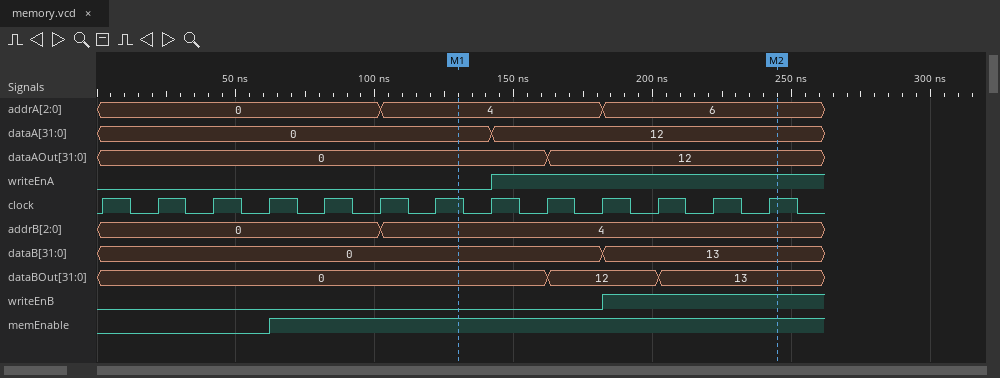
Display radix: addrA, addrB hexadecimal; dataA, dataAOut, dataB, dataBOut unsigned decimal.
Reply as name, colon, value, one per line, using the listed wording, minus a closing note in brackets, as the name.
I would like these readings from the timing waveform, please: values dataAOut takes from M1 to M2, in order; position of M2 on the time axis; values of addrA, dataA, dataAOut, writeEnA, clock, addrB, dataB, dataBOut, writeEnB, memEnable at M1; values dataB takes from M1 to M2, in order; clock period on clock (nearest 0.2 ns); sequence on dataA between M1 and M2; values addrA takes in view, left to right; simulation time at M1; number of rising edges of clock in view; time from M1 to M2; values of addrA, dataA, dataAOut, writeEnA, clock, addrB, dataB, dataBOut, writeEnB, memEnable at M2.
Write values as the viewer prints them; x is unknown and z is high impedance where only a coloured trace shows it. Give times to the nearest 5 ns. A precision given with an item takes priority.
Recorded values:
values dataAOut takes from M1 to M2, in order: 0, 12
position of M2 on the time axis: 245 ns
values of addrA, dataA, dataAOut, writeEnA, clock, addrB, dataB, dataBOut, writeEnB, memEnable at M1: addrA=4, dataA=0, dataAOut=0, writeEnA=0, clock=1, addrB=4, dataB=0, dataBOut=0, writeEnB=0, memEnable=1
values dataB takes from M1 to M2, in order: 0, 13
clock period on clock: 20 ns
sequence on dataA between M1 and M2: 0, 12
values addrA takes in view, left to right: 0, 4, 6
simulation time at M1: 130 ns
number of rising edges of clock in view: 13
time from M1 to M2: 115 ns
values of addrA, dataA, dataAOut, writeEnA, clock, addrB, dataB, dataBOut, writeEnB, memEnable at M2: addrA=6, dataA=12, dataAOut=12, writeEnA=1, clock=1, addrB=4, dataB=13, dataBOut=13, writeEnB=1, memEnable=1
